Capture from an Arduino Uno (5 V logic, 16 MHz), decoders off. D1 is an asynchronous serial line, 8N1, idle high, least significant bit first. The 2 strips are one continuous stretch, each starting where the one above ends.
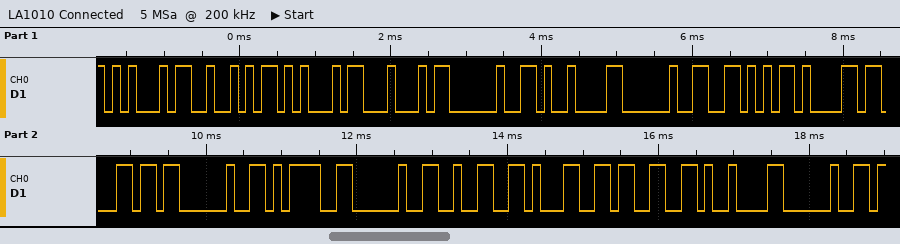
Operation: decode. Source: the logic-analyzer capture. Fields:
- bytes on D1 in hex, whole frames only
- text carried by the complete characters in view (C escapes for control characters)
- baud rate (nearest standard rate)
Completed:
45 52 45 44 20 09 20 56 61 6C 20 3D 20 32 31 33 09 20
"ERED \t Val = 213\t "
9600 baud
